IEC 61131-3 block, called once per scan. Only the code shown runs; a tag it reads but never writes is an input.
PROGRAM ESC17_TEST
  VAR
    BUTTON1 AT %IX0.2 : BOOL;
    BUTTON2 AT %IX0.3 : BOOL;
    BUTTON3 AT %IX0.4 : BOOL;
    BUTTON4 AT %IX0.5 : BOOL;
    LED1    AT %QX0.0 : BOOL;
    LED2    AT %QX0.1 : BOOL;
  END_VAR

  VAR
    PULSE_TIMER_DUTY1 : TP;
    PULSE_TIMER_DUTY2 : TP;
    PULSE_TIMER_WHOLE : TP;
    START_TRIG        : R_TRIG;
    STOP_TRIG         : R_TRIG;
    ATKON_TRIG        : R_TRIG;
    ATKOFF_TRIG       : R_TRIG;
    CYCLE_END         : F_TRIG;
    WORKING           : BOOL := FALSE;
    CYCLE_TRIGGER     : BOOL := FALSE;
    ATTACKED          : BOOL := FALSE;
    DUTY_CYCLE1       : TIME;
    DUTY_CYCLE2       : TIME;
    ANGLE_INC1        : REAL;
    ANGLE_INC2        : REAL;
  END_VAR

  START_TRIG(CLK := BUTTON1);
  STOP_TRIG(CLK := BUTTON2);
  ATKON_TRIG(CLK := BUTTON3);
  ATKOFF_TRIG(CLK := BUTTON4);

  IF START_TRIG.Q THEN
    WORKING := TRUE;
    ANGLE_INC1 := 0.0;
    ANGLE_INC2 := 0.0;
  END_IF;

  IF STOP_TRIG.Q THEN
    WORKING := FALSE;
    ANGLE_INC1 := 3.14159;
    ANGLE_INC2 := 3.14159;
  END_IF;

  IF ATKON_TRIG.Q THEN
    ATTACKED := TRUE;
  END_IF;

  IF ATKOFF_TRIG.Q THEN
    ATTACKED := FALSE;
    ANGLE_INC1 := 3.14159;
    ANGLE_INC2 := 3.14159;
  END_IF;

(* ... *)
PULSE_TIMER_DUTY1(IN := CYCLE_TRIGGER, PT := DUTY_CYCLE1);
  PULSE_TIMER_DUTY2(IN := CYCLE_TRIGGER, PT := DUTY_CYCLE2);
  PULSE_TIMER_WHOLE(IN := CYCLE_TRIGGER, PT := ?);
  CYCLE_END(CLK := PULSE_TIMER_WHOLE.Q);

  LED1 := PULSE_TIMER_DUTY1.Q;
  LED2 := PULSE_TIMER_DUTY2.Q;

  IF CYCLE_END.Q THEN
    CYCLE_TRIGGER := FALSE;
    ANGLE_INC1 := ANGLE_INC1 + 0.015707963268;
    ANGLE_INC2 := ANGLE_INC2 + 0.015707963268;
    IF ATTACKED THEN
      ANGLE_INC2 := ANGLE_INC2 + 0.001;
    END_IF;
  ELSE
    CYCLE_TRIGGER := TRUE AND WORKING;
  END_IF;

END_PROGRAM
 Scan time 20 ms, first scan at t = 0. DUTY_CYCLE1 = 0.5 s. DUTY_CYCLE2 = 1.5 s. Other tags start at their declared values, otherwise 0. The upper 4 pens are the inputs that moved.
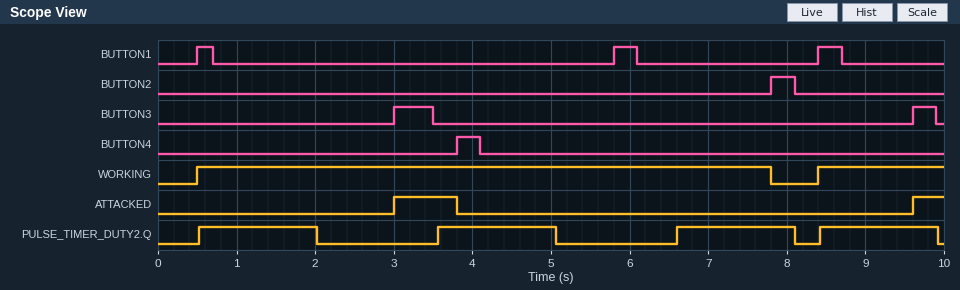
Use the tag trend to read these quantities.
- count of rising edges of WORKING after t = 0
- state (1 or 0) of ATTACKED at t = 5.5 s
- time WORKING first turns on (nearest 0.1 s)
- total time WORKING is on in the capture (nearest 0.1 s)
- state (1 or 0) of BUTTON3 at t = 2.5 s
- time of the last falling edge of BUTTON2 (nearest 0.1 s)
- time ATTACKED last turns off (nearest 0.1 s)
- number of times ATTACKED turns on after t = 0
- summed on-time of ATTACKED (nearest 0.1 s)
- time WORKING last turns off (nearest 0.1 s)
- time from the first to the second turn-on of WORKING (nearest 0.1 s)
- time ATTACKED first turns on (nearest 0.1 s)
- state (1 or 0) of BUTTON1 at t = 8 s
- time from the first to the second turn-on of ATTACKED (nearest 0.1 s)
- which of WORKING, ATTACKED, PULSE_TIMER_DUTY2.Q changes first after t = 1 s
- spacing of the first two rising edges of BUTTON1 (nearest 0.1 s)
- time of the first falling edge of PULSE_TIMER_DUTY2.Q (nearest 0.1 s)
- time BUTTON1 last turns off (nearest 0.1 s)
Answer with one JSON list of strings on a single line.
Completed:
["2", "0", "0.5 s", "8.9 s", "0", "8.1 s", "3.8 s", "2", "1.2 s", "7.8 s", "7.9 s", "3.0 s", "0", "6.6 s", "PULSE_TIMER_DUTY2.Q", "5.3 s", "2.0 s", "8.7 s"]
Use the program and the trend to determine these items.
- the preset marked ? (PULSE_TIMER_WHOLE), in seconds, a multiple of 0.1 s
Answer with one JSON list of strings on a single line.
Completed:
["3.0 s"]
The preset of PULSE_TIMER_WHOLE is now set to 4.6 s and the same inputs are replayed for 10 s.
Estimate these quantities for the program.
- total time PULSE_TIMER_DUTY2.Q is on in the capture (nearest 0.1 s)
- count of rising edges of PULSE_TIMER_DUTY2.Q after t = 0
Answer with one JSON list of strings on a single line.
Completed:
["4.5 s", "3"]
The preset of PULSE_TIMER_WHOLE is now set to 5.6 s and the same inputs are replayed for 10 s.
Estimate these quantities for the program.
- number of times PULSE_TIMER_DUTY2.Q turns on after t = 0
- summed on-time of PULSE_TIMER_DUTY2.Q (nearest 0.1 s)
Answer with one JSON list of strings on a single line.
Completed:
["3", "4.5 s"]
